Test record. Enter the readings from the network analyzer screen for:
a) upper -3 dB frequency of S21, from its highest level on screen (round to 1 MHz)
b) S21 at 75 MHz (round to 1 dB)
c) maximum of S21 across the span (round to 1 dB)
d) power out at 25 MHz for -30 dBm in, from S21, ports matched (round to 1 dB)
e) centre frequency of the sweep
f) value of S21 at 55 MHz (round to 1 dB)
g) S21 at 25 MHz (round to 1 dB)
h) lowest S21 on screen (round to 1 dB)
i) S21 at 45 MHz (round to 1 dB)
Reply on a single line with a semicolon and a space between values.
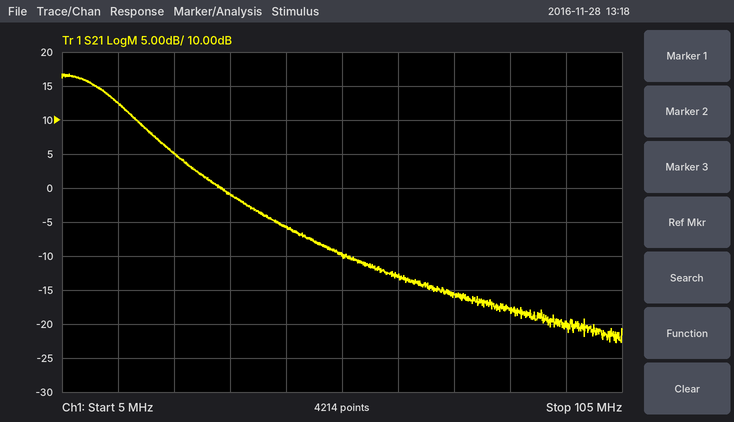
13 MHz; -16 dB; 17 dB; -25 dBm; 55 MHz; -10 dB; 5 dB; -23 dB; -6 dB
